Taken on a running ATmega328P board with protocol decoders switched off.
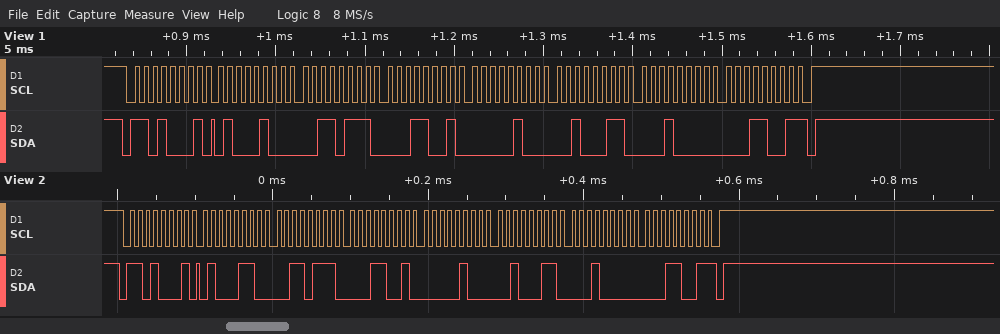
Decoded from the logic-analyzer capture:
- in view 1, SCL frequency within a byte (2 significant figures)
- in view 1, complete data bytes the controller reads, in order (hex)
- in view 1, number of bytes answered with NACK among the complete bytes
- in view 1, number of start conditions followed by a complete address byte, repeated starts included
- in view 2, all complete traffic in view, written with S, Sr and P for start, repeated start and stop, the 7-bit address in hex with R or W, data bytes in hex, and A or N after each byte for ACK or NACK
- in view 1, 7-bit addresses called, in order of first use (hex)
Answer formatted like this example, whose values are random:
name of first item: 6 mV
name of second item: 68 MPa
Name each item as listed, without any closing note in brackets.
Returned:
in view 1, SCL frequency within a byte: 100 kHz
in view 1, complete data bytes the controller reads, in order: 44 37 19 04 23 10 19
in view 1, number of bytes answered with NACK among the complete bytes: 1
in view 1, number of start conditions followed by a complete address byte, repeated starts included: 1
in view 2, all complete traffic in view, written with S, Sr and P for start, repeated start and stop, the 7-bit address in hex with R or W, data bytes in hex, and A or N after each byte for ACK or NACK: S 68R A 46 A 37 A 19 A 04 A 23 A 10 A 19 N P
in view 1, 7-bit addresses called, in order of first use: 0x68
